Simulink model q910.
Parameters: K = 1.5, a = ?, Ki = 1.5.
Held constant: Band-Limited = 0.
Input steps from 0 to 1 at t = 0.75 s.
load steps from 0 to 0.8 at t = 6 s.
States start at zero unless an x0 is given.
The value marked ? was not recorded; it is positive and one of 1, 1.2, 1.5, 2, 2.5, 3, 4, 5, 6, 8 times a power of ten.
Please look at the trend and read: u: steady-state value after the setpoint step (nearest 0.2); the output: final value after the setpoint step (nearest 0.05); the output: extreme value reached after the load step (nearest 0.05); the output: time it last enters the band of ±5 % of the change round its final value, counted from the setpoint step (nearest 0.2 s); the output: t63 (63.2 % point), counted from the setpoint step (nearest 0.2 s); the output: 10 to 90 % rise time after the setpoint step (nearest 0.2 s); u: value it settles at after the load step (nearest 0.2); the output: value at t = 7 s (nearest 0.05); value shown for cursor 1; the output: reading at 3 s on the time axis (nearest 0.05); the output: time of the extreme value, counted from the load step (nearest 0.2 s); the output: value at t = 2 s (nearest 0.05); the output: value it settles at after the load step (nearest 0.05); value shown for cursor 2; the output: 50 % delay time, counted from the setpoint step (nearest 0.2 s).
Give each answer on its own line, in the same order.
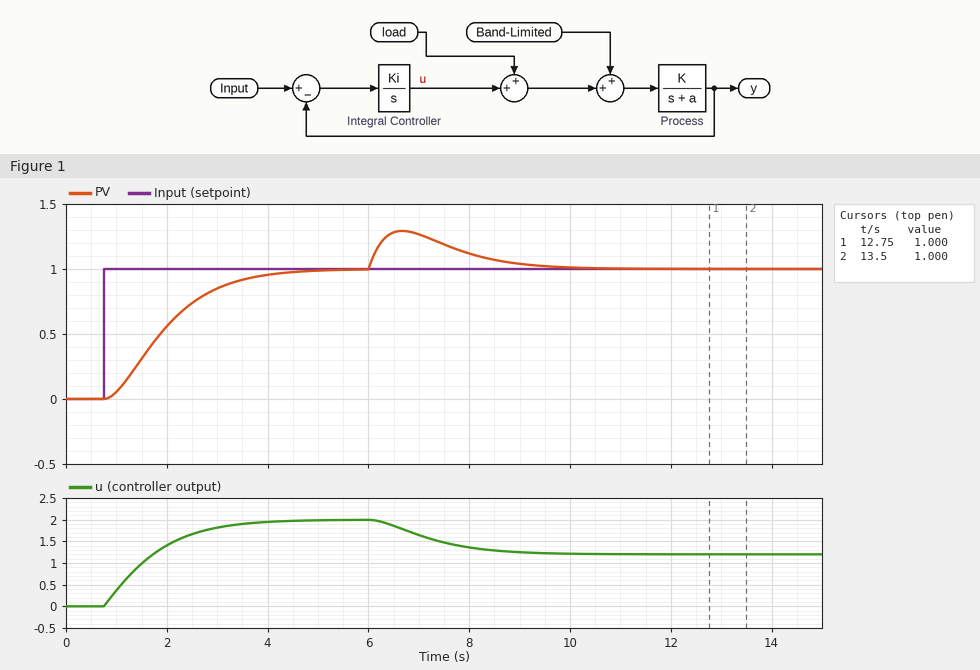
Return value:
2.0
1.00
1.30
3.2 s
1.4 s
2.2 s
1.2
1.25
1.000
0.85
0.6 s
0.55
1.00
1.000
1.2 s
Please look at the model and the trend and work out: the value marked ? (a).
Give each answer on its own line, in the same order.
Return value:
3
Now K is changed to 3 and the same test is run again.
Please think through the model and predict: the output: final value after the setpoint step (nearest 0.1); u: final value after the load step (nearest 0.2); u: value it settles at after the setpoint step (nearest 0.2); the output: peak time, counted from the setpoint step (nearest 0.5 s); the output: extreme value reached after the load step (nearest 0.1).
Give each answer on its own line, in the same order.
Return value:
1.0
0.2
1.0
2.0 s
1.5
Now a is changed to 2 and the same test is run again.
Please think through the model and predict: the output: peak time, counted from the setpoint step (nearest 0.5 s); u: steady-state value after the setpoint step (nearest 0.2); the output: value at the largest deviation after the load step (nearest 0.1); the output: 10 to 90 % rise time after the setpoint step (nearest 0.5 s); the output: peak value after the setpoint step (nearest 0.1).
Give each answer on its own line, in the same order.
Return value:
3.0 s
1.4
1.4
1.5 s
1.1
